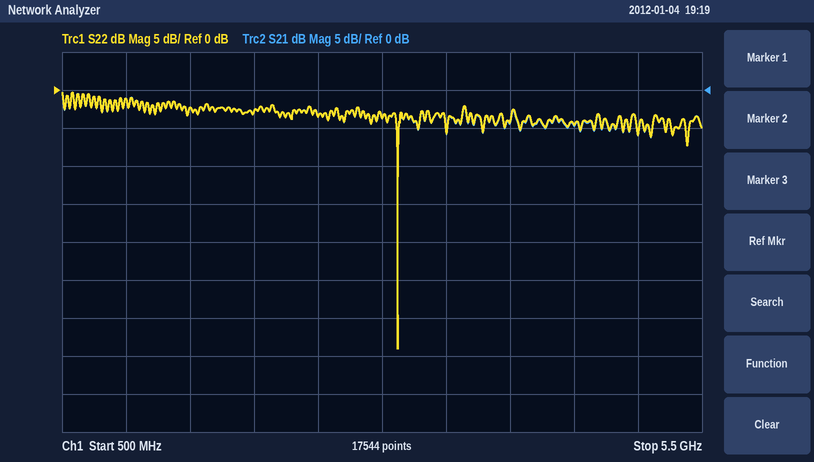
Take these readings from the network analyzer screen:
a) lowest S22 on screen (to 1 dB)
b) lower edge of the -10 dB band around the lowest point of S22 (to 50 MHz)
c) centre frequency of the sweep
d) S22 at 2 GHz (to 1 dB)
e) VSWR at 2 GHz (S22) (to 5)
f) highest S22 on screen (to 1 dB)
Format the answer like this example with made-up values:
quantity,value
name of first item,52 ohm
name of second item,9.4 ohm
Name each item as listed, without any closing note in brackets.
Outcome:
quantity,value
lowest S22 on screen,-34 dB
lower edge of the -10 dB band around the lowest point of S22,3.10 GHz
centre frequency of the sweep,3 GHz
S22 at 2 GHz,-3 dB
VSWR at 2 GHz (S22),5
highest S22 on screen,0 dB
